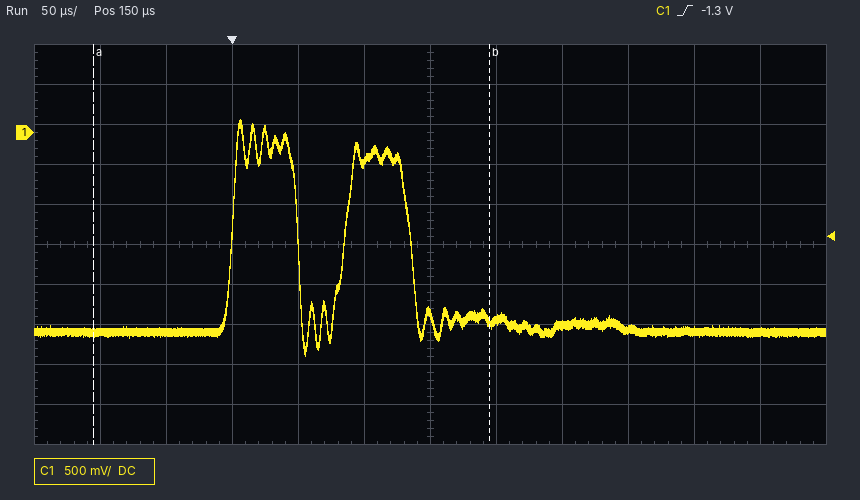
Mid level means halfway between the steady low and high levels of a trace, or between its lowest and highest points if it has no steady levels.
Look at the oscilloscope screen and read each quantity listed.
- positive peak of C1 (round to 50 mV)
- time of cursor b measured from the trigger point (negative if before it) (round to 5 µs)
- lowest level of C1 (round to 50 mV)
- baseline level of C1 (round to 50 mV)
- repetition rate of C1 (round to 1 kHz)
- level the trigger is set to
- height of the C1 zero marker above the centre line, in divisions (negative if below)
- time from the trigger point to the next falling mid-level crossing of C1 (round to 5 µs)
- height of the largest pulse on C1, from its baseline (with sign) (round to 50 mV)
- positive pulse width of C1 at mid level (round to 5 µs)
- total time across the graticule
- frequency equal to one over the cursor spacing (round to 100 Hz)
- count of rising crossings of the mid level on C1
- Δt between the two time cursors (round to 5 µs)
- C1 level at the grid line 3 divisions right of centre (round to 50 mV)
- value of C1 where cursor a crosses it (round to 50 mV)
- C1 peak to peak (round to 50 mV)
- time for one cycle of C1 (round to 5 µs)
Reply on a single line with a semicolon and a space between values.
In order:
150 mV; +195 µs; -2.80 V; -2.50 V; 12 kHz; -1.3 V; +2.8 div; 50 µs; +2.65 V; 50 µs; 600 µs; 3.3 kHz; 2; 300 µs; -2.45 V; -2.50 V; 2.95 V; 85 µs
